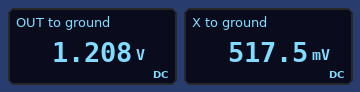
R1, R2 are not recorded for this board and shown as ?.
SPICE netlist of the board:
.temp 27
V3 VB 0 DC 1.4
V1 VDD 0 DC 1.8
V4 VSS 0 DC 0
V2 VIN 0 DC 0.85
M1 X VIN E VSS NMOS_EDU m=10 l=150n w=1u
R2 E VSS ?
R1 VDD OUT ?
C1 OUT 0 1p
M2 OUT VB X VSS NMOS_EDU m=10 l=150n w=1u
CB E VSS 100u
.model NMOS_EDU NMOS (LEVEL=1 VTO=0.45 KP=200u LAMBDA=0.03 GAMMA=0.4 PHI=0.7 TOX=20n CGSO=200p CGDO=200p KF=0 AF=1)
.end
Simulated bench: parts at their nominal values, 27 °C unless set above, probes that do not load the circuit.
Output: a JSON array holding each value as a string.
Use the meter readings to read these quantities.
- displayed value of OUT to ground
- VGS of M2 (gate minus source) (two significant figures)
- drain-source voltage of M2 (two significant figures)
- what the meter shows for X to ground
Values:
["1.208 V", "880 mV", "690 mV", "517.5 mV"]
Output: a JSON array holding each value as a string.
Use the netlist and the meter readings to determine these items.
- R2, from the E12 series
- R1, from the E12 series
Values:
["82 Ω", "820 Ω"]
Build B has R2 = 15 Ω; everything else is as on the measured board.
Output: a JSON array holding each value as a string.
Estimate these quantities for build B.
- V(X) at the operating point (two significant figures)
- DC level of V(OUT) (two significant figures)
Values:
["470 mV", "990 mV"]
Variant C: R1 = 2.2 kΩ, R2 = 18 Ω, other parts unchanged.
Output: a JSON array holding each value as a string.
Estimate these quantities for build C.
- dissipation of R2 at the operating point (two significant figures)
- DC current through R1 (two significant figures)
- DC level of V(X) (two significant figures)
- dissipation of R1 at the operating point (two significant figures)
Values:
["8.8 µW", "700 µA", "190 mV", "1.1 mW"]
